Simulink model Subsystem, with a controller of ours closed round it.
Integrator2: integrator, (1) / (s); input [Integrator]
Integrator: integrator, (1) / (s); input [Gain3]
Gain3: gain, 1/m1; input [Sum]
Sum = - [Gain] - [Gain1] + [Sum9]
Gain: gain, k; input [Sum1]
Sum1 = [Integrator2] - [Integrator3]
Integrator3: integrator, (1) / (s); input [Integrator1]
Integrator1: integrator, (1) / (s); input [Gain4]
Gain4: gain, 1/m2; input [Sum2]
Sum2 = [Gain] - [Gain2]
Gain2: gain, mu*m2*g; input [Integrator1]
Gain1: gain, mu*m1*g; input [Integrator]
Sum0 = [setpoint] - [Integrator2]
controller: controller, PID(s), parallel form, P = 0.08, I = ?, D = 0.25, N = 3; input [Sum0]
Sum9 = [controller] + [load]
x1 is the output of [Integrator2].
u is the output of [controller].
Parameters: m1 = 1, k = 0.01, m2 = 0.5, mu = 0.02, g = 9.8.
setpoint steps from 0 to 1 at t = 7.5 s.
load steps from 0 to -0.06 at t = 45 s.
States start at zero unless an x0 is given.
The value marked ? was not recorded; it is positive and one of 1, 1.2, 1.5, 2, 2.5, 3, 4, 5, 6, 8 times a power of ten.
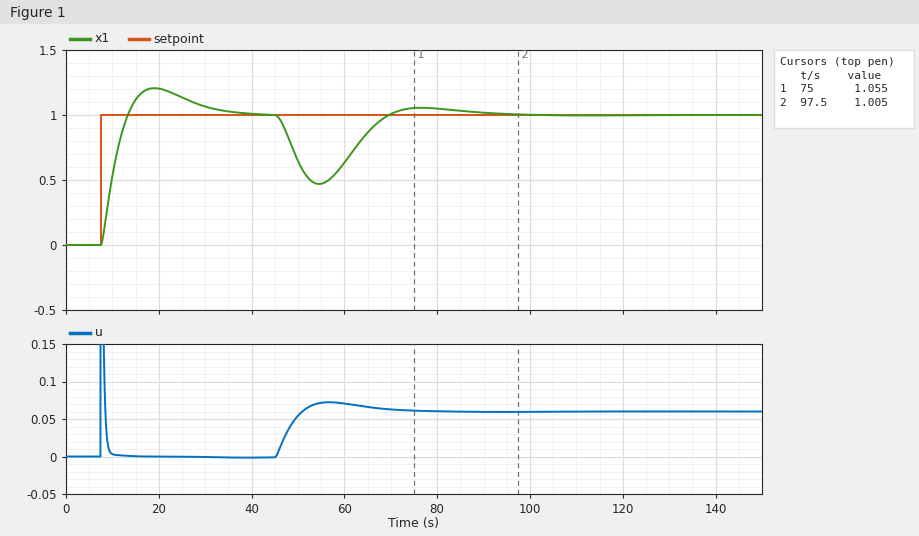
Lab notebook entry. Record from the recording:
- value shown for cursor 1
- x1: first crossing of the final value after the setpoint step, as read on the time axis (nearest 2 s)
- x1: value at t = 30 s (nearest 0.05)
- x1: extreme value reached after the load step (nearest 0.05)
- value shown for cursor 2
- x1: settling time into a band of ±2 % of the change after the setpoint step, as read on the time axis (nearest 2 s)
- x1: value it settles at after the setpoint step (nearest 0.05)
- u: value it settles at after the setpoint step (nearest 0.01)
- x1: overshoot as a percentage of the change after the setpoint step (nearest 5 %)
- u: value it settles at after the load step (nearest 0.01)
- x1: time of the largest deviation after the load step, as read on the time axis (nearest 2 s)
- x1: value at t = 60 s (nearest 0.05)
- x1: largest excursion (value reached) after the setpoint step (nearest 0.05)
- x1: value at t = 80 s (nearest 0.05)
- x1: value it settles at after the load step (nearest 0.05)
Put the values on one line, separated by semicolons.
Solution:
1.055; 14 s; 1.05; 0.45; 1.005; 36 s; 1.00; 0.00; 20 %; 0.06; 54 s; 0.65; 1.20; 1.05; 1.00
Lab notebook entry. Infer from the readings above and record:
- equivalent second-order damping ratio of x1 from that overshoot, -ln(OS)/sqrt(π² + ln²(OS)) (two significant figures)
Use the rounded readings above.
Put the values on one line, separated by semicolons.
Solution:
0.46
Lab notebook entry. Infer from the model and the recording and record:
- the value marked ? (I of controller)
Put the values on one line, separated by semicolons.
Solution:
0.01
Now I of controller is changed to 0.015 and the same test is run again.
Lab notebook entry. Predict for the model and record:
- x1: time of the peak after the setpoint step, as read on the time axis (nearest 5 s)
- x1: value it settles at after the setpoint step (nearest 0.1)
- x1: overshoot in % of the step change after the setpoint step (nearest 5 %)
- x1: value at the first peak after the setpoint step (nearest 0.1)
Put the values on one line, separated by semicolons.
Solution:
20 s; 1.0; 30 %; 1.3
